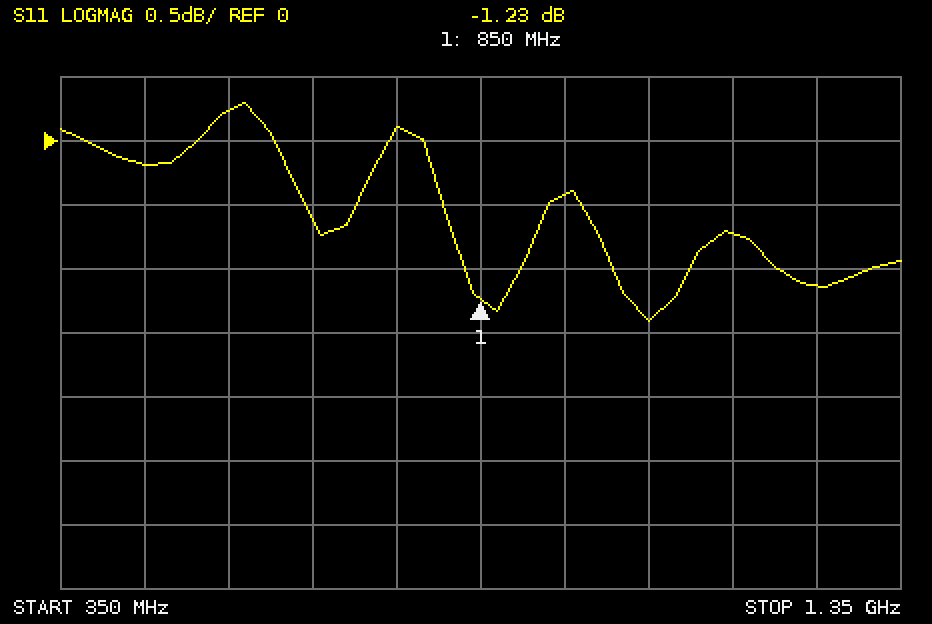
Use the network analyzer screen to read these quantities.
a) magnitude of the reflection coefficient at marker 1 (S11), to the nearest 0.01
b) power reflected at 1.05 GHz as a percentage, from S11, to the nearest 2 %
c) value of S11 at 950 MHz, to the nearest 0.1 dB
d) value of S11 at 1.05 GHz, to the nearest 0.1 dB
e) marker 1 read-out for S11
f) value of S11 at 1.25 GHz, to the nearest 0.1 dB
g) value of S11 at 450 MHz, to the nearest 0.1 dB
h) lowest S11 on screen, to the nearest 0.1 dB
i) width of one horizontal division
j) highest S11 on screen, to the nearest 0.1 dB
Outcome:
0.87
72 %
-0.4 dB
-1.4 dB
-1.23 dB
-1.1 dB
-0.2 dB
-1.4 dB
100 MHz
0.3 dB
